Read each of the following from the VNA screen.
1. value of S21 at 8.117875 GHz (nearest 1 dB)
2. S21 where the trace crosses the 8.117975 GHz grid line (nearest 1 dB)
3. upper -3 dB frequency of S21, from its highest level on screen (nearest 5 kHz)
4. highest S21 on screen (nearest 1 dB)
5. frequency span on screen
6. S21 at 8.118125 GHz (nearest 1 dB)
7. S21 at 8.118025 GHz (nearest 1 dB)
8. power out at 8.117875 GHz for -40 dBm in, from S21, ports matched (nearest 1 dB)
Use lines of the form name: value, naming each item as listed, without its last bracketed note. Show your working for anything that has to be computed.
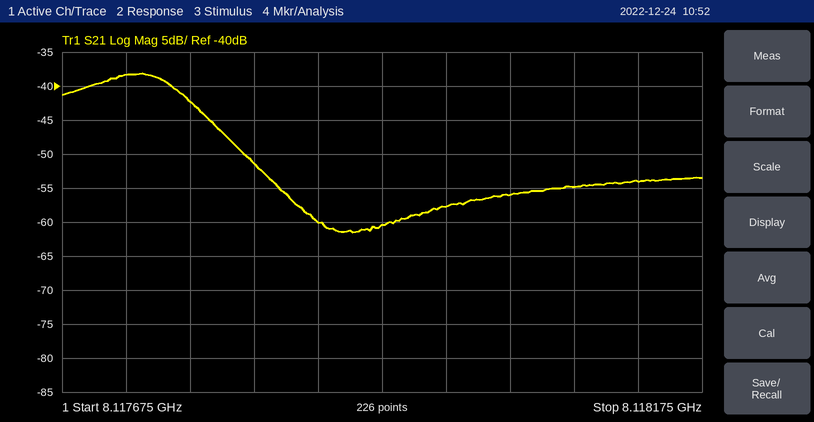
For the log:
value of S21 at 8.117875 GHz: -60 dB
S21 where the trace crosses the 8.117975 GHz grid line: -58 dB
upper -3 dB frequency of S21, from its highest level on screen: 8.117770 GHz
highest S21 on screen: -38 dB
frequency span on screen: 500 kHz
S21 at 8.118125 GHz: -54 dB
S21 at 8.118025 GHz: -56 dB
power out at 8.117875 GHz for -40 dBm in, from S21, ports matched: -40 dBm + (-60 dB) = -100 dBm
